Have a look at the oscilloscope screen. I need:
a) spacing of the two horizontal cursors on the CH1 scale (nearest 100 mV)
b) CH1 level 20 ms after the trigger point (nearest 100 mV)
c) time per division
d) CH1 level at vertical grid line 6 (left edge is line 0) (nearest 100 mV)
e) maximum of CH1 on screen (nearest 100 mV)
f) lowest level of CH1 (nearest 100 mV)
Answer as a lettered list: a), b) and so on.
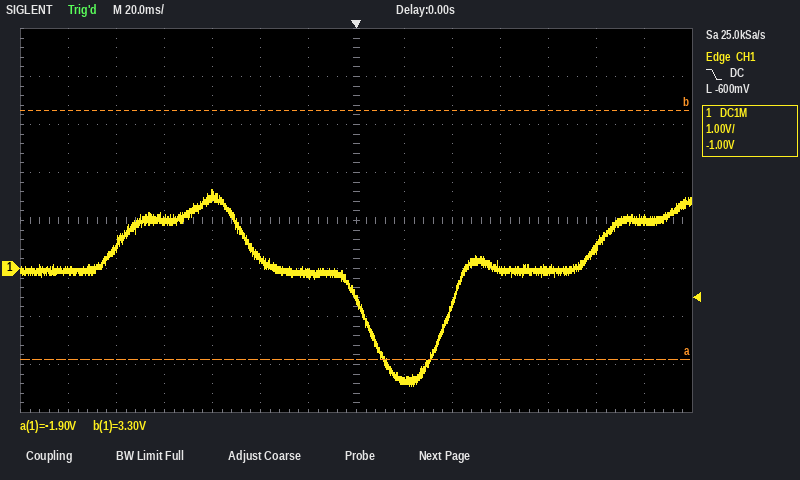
a) 5.2 V
b) -2.3 V
c) 20 ms
d) -100 mV
e) 1.6 V
f) -2.4 V
